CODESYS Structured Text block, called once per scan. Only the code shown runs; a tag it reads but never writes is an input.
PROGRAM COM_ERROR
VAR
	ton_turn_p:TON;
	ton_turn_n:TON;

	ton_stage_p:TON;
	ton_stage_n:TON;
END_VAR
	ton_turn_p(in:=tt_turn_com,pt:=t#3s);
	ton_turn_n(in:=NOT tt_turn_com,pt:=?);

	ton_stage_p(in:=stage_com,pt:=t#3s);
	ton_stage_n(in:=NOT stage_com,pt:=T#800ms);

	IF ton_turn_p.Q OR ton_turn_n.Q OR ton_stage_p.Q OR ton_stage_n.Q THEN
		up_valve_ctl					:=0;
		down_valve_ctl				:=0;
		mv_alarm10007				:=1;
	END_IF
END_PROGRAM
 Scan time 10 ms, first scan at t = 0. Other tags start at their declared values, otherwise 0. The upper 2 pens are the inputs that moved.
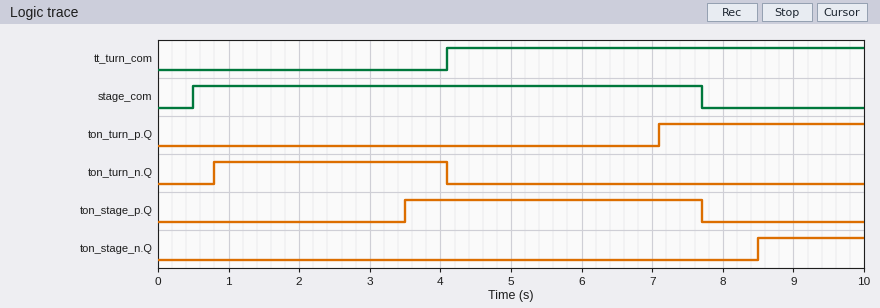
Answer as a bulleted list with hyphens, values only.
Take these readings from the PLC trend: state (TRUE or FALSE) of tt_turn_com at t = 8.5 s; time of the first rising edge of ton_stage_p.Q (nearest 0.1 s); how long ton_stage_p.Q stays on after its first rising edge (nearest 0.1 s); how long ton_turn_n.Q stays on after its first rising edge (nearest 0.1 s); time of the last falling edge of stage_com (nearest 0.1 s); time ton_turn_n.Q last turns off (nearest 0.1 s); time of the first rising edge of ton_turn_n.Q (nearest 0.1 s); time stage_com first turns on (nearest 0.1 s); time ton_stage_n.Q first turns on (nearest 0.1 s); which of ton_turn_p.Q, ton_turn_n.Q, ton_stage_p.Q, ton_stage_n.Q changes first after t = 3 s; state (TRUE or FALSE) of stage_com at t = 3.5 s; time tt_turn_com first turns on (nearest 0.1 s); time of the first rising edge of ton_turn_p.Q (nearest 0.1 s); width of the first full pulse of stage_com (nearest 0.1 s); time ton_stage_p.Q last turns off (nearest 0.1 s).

- TRUE
- 3.5 s
- 4.2 s
- 3.3 s
- 7.7 s
- 4.1 s
- 0.8 s
- 0.5 s
- 8.5 s
- ton_stage_p.Q
- TRUE
- 4.1 s
- 7.1 s
- 7.2 s
- 7.7 s
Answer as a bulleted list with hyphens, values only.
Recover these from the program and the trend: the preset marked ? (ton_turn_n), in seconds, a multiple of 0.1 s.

- 0.8 s
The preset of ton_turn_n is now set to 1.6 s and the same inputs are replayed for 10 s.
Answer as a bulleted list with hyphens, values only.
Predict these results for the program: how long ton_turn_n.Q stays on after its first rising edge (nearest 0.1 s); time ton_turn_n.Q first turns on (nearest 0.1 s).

- 2.5 s
- 1.6 s
